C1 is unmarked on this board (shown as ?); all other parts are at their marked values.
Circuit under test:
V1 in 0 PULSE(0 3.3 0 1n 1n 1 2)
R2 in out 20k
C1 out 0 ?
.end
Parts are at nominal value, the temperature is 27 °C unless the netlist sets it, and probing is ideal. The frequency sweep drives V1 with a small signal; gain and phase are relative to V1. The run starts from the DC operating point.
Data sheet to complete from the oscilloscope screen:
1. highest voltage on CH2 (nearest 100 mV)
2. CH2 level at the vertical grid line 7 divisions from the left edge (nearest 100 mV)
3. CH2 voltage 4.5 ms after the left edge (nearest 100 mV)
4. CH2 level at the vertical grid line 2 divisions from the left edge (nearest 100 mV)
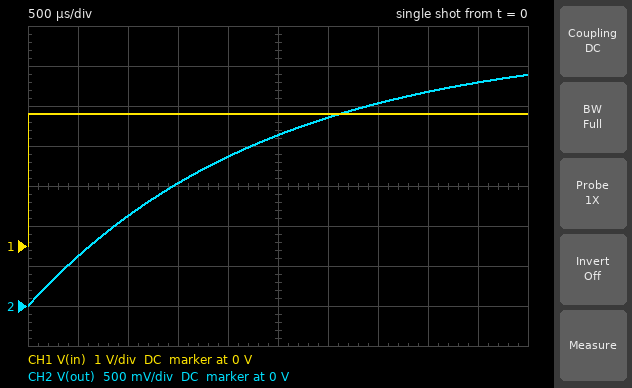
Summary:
2.9 V
2.5 V
2.8 V
1.1 V
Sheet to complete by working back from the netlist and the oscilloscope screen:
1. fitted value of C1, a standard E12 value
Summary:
120 nF
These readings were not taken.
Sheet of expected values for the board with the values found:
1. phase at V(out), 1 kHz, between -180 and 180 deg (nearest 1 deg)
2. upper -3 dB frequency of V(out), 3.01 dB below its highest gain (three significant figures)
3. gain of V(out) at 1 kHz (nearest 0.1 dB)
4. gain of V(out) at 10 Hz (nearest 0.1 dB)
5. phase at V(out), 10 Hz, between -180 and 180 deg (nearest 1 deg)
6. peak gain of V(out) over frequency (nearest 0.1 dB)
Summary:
-86 deg
66.3 Hz
-23.6 dB
-0.1 dB
-9 deg
0 dB
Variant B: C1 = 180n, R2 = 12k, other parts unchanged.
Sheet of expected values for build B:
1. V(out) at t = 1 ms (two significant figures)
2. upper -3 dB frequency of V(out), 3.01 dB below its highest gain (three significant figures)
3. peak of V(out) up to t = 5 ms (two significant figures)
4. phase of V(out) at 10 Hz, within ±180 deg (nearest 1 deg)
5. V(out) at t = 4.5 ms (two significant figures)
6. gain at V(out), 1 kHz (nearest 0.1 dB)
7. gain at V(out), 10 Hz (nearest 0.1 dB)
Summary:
1.2 V
73.7 Hz
3.0 V
-8 deg
2.9 V
-22.7 dB
-0.1 dB
